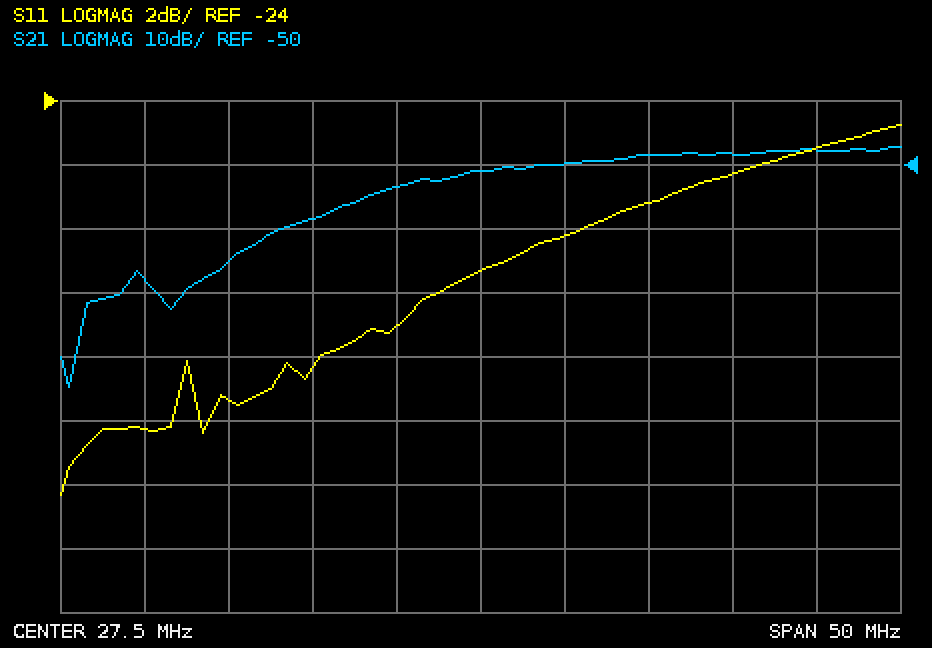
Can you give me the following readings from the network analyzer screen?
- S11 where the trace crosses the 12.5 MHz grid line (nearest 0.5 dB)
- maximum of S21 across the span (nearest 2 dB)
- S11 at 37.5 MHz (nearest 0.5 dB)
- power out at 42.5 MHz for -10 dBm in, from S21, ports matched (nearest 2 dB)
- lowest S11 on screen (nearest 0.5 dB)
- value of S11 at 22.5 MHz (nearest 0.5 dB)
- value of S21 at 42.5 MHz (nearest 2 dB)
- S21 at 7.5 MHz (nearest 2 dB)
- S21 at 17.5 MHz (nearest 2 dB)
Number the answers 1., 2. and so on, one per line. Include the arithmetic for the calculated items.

1. -33.5 dB
2. -48 dB
3. -27.0 dB
4. -10 dBm + (-48 dB) = -58 dBm
5. -36.5 dB
6. -31.0 dB
7. -48 dB
8. -68 dB
9. -58 dB
